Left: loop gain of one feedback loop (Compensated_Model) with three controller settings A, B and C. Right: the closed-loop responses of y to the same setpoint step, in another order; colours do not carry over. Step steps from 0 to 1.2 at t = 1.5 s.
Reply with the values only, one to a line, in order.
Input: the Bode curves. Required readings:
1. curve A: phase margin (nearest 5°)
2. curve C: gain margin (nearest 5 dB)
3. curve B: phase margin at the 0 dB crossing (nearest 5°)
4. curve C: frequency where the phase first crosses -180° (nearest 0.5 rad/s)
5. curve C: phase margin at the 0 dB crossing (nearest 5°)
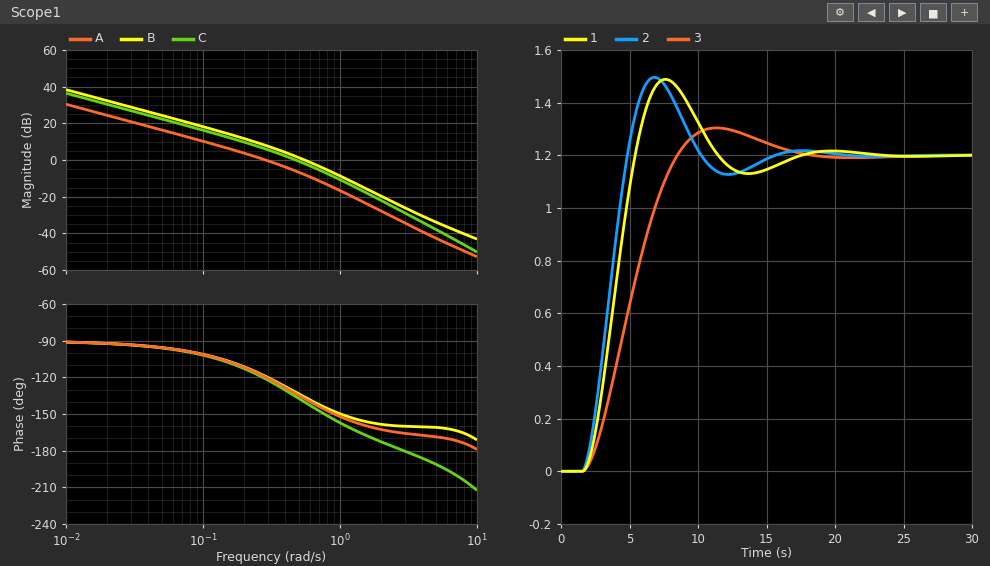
60°
30 dB
45°
3.0 rad/s
45°
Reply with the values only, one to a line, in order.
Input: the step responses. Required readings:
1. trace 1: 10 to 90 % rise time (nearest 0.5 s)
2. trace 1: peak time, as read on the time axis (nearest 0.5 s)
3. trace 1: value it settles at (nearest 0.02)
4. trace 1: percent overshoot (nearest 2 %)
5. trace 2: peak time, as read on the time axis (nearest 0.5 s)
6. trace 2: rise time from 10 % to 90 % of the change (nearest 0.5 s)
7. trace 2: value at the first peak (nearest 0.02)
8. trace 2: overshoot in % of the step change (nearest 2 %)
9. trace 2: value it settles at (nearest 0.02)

2.5 s
7.5 s
1.20
24 %
7.0 s
2.5 s
1.50
24 %
1.20
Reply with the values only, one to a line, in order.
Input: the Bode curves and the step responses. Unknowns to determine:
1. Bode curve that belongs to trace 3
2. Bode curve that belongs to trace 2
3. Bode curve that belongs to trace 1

A
B
C
